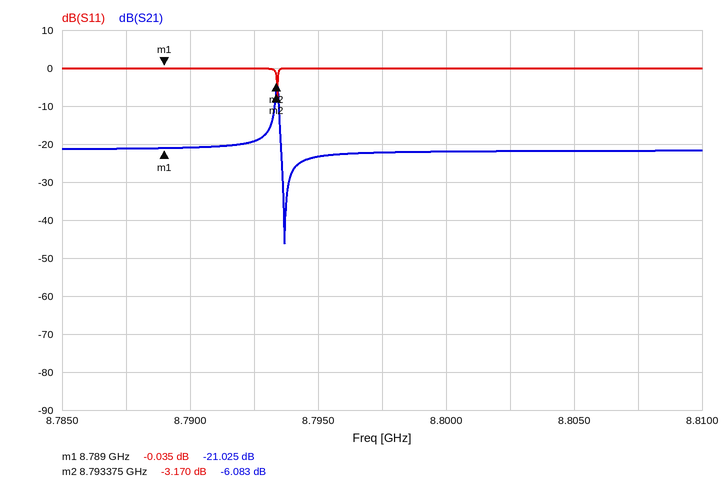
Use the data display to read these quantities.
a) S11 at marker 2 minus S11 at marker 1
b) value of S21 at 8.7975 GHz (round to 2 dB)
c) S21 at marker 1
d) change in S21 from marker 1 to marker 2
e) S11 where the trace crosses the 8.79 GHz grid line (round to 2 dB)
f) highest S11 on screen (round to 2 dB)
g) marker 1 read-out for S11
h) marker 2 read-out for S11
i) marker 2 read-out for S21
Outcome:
-3.135 dB
-22 dB
-21.025 dB
14.942 dB
0 dB
0 dB
-0.035 dB
-3.170 dB
-6.083 dB
